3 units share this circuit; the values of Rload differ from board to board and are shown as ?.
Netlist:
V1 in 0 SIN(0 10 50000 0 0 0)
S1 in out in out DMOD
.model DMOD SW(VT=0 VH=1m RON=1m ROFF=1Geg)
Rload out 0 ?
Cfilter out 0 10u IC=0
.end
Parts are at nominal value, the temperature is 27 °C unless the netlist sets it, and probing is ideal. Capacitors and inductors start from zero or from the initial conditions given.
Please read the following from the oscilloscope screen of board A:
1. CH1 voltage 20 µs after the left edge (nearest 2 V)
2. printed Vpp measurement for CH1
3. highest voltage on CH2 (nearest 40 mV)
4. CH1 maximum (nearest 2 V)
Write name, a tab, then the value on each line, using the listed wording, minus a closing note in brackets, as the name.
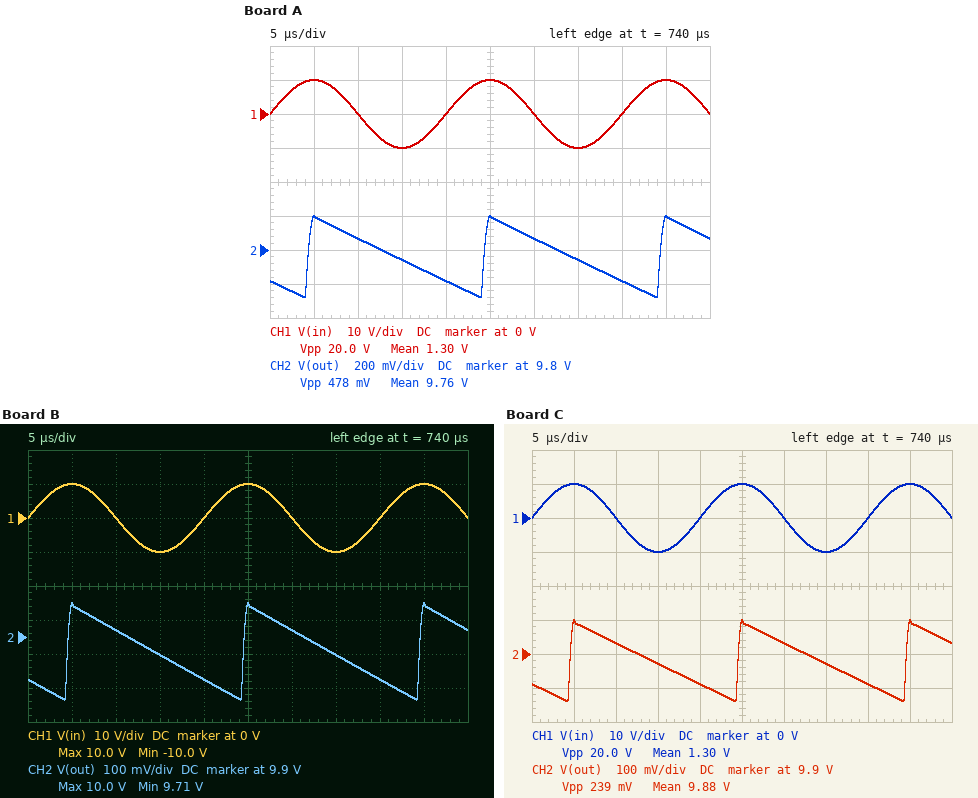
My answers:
CH1 voltage 20 µs after the left edge	0 V
printed Vpp measurement for CH1	20.0 V
highest voltage on CH2	10.00 V
CH1 maximum	10 V
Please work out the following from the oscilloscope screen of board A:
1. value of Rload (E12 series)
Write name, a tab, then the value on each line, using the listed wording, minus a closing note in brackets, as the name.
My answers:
value of Rload	39 Ω
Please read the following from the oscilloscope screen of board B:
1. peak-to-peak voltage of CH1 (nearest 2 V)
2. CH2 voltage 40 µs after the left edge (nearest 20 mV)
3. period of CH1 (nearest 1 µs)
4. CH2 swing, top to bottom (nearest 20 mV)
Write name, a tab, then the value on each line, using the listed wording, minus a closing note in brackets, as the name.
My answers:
peak-to-peak voltage of CH1	20 V
CH2 voltage 40 µs after the left edge	9.78 V
period of CH1	20 µs
CH2 swing, top to bottom	280 mV
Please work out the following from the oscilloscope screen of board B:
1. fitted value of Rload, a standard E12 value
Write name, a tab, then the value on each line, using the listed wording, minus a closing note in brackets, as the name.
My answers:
fitted value of Rload, a standard E12 value	68 Ω
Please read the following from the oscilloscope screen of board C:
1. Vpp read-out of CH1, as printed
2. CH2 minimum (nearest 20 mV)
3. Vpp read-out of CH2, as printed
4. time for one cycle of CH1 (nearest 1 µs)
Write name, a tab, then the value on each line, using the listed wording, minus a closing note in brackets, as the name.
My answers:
Vpp read-out of CH1, as printed	20.0 V
CH2 minimum	9.76 V
Vpp read-out of CH2, as printed	239 mV
time for one cycle of CH1	20 µs
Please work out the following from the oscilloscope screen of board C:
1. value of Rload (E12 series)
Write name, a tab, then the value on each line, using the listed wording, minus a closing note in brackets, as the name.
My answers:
value of Rload	82 Ω
